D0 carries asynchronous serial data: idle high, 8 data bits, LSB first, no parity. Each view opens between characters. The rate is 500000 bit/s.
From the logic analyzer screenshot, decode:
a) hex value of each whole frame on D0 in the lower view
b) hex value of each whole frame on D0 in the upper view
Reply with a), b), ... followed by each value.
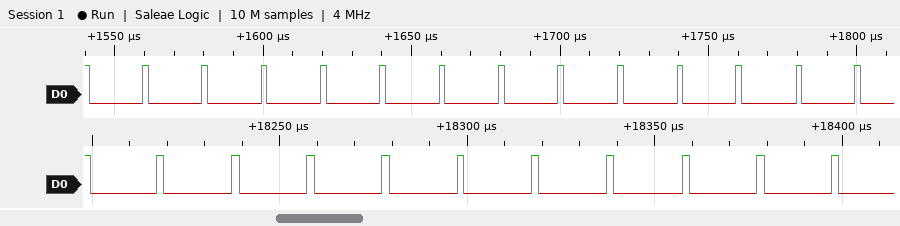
a) 00, 00, 00, 00, 00, 00, 00, 00, 00, 00
b) 00, 00, 00, 00, 00, 00, 00, 00, 00, 00, 00, 00, 00
